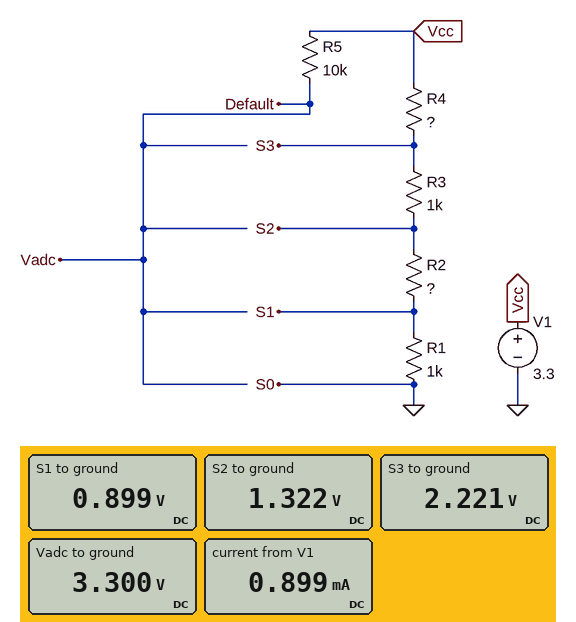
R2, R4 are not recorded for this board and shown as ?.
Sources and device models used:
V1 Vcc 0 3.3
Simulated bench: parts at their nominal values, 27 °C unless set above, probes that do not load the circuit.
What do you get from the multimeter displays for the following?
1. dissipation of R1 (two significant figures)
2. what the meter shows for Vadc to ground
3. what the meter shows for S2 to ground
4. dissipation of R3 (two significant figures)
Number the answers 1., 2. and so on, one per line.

1. 810 µW
2. 3.300 V
3. 1.322 V
4. 810 µW
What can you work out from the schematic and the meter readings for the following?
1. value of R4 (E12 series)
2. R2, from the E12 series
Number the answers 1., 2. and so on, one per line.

1. 1.2 kΩ
2. 470 Ω
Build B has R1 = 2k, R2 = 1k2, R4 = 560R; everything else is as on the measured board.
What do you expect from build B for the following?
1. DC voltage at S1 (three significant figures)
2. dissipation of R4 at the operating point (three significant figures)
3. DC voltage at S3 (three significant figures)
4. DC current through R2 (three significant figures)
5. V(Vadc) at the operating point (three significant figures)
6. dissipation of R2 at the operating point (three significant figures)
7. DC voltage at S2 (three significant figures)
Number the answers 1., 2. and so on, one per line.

1. 1.39 V
2. 269 µW
3. 2.91 V
4. 693 µA
5. 3.30 V
6. 577 µW
7. 2.22 V
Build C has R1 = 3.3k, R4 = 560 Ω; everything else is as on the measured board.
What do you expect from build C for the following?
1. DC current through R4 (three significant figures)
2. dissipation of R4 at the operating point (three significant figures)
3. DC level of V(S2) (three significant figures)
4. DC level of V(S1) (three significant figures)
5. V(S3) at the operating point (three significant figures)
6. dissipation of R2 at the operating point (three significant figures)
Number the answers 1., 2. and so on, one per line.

1. 619 µA
2. 215 µW
3. 2.33 V
4. 2.04 V
5. 2.95 V
6. 180 µW
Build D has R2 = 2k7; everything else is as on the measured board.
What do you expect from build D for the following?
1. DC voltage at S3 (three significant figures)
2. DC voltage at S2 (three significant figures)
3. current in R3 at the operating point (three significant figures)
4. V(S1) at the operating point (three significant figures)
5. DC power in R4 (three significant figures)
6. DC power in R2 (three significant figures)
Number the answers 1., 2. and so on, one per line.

1. 2.63 V
2. 2.07 V
3. 559 µA
4. 559 mV
5. 375 µW
6. 845 µW
